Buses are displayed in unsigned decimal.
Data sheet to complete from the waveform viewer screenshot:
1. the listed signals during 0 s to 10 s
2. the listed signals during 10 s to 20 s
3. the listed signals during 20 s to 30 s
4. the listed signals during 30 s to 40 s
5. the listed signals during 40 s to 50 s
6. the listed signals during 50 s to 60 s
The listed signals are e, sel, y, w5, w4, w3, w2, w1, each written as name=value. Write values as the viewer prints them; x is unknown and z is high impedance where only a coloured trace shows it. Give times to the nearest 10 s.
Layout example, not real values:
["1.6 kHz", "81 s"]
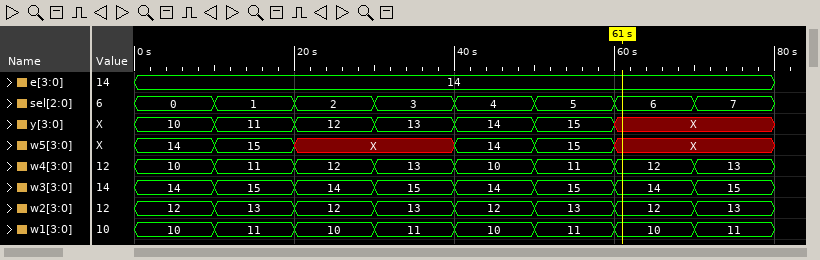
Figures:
["e=14, sel=0, y=10, w5=14, w4=10, w3=14, w2=12, w1=10", "e=14, sel=1, y=11, w5=15, w4=11, w3=15, w2=13, w1=11", "e=14, sel=2, y=12, w5=X, w4=12, w3=14, w2=12, w1=10", "e=14, sel=3, y=13, w5=X, w4=13, w3=15, w2=13, w1=11", "e=14, sel=4, y=14, w5=14, w4=10, w3=14, w2=12, w1=10", "e=14, sel=5, y=15, w5=15, w4=11, w3=15, w2=13, w1=11"]
